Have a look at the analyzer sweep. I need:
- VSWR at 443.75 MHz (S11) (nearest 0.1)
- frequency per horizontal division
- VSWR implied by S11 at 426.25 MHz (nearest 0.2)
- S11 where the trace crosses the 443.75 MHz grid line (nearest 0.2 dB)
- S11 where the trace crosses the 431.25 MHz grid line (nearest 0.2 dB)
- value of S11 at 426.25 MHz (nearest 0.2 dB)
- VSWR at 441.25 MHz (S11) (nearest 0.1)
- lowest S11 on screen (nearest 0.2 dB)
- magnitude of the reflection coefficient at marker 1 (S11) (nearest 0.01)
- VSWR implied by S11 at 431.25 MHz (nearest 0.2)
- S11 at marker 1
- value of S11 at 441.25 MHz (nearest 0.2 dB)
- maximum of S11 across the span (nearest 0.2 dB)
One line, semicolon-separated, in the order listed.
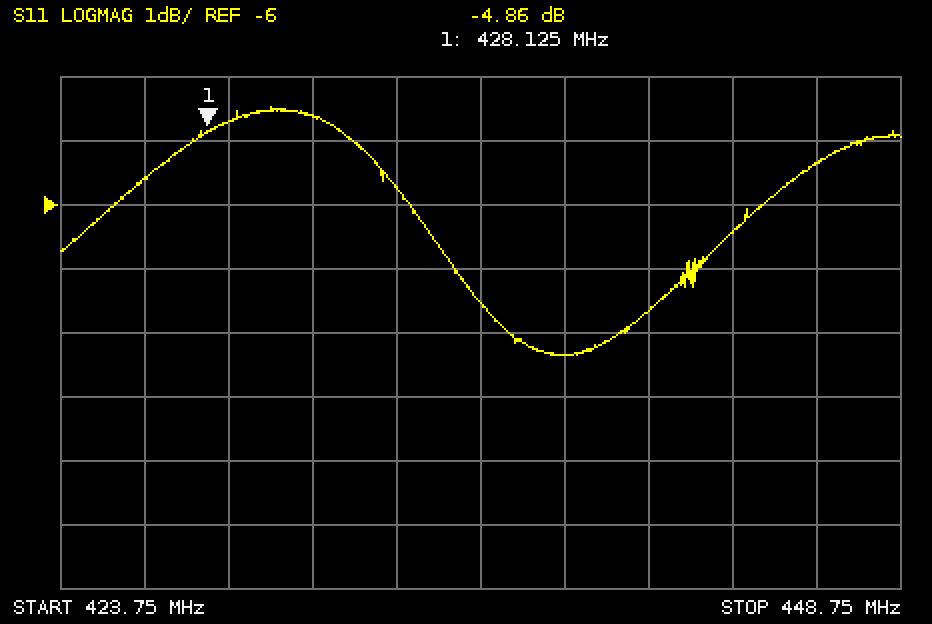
2.8; 2.5 MHz; 3.2; -6.4 dB; -4.6 dB; -5.6 dB; 2.4; -8.4 dB; 0.57; 3.8; -4.86 dB; -7.6 dB; -4.4 dB
